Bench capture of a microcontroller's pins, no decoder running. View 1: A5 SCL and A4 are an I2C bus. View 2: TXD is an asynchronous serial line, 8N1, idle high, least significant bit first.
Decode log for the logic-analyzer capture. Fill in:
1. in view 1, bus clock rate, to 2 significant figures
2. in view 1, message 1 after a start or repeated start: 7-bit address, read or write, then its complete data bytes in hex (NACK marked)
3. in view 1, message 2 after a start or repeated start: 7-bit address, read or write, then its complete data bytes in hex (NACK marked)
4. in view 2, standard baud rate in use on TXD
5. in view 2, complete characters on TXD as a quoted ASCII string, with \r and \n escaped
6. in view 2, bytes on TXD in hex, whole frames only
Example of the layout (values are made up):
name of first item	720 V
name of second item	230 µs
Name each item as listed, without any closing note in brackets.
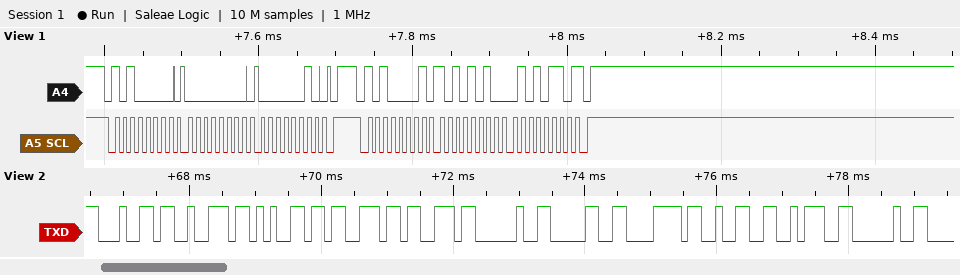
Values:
in view 1, bus clock rate, to 2 significant figures	100 kHz
in view 1, message 1 after a start or repeated start: 7-bit address, read or write, then its complete data bytes in hex	0x50 write: 00 02
in view 1, message 2 after a start or repeated start: 7-bit address, read or write, then its complete data bytes in hex	0x50 read: AA 56 NACK
in view 2, standard baud rate in use on TXD	9600 baud
in view 2, complete characters on TXD as a quoted ASCII string, with \r and \n escaped	"dress 0x2: "
in view 2, bytes on TXD in hex, whole frames only	64 72 65 73 73 20 30 78 32 3A 20
